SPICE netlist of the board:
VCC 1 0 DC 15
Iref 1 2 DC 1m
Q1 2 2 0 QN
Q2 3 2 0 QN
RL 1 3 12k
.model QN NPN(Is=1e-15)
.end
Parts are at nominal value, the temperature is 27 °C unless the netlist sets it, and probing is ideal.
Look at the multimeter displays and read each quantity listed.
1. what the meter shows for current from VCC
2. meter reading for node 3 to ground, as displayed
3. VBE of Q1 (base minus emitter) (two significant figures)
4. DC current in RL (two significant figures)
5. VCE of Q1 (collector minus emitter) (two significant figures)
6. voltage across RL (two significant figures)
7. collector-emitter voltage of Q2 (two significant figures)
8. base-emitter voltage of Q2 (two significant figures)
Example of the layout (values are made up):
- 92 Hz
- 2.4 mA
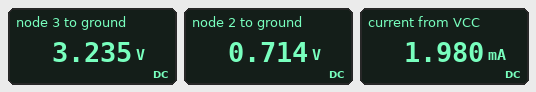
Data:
- 1.980 mA
- 3.235 V
- 710 mV
- 980 µA
- 710 mV
- 12 V
- 3.2 V
- 710 mV
